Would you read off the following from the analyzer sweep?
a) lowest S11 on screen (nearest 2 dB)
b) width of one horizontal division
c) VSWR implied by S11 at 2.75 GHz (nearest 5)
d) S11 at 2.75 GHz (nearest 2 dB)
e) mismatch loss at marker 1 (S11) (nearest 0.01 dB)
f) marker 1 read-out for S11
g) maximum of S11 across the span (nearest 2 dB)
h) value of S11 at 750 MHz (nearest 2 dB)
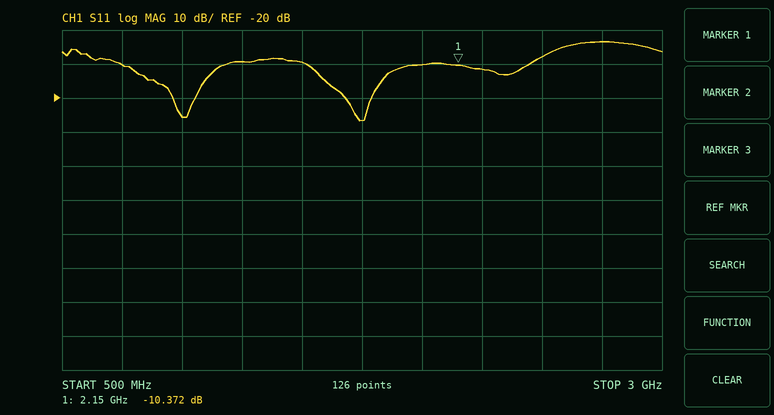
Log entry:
-26 dB
250 MHz
5
-4 dB
0.42 dB
-10.372 dB
-4 dB
-10 dB
